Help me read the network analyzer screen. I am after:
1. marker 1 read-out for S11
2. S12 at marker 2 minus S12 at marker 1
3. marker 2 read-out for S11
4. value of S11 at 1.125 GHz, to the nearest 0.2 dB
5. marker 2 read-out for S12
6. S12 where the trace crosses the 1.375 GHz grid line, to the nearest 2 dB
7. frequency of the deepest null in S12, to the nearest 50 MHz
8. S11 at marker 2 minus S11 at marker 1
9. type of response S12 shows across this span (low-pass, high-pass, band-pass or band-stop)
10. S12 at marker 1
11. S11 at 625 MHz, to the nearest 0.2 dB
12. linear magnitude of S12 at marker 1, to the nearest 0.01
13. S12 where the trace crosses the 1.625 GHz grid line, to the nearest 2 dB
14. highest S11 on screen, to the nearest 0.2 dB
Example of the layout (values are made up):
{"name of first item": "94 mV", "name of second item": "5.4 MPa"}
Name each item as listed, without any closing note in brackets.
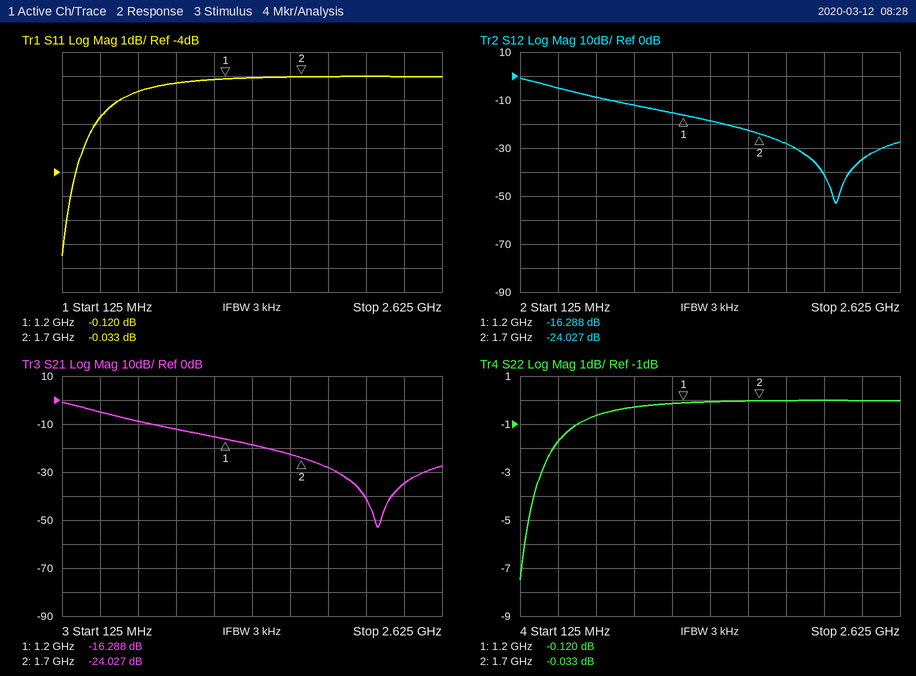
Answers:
{"marker 1 read-out for S11": "-0.120 dB", "S12 at marker 2 minus S12 at marker 1": "-7.739 dB", "marker 2 read-out for S11": "-0.033 dB", "value of S11 at 1.125 GHz, to the nearest 0.2 dB": "-0.2 dB", "marker 2 read-out for S12": "-24.027 dB", "S12 where the trace crosses the 1.375 GHz grid line, to the nearest 2 dB": "-18 dB", "frequency of the deepest null in S12, to the nearest 50 MHz": "2.20 GHz", "S11 at marker 2 minus S11 at marker 1": "0.087 dB", "type of response S12 shows across this span": "low-pass", "S12 at marker 1": "-16.288 dB", "S11 at 625 MHz, to the nearest 0.2 dB": "-0.6 dB", "linear magnitude of S12 at marker 1, to the nearest 0.01": "0.15", "S12 where the trace crosses the 1.625 GHz grid line, to the nearest 2 dB": "-22 dB", "highest S11 on screen, to the nearest 0.2 dB": "0.0 dB"}
